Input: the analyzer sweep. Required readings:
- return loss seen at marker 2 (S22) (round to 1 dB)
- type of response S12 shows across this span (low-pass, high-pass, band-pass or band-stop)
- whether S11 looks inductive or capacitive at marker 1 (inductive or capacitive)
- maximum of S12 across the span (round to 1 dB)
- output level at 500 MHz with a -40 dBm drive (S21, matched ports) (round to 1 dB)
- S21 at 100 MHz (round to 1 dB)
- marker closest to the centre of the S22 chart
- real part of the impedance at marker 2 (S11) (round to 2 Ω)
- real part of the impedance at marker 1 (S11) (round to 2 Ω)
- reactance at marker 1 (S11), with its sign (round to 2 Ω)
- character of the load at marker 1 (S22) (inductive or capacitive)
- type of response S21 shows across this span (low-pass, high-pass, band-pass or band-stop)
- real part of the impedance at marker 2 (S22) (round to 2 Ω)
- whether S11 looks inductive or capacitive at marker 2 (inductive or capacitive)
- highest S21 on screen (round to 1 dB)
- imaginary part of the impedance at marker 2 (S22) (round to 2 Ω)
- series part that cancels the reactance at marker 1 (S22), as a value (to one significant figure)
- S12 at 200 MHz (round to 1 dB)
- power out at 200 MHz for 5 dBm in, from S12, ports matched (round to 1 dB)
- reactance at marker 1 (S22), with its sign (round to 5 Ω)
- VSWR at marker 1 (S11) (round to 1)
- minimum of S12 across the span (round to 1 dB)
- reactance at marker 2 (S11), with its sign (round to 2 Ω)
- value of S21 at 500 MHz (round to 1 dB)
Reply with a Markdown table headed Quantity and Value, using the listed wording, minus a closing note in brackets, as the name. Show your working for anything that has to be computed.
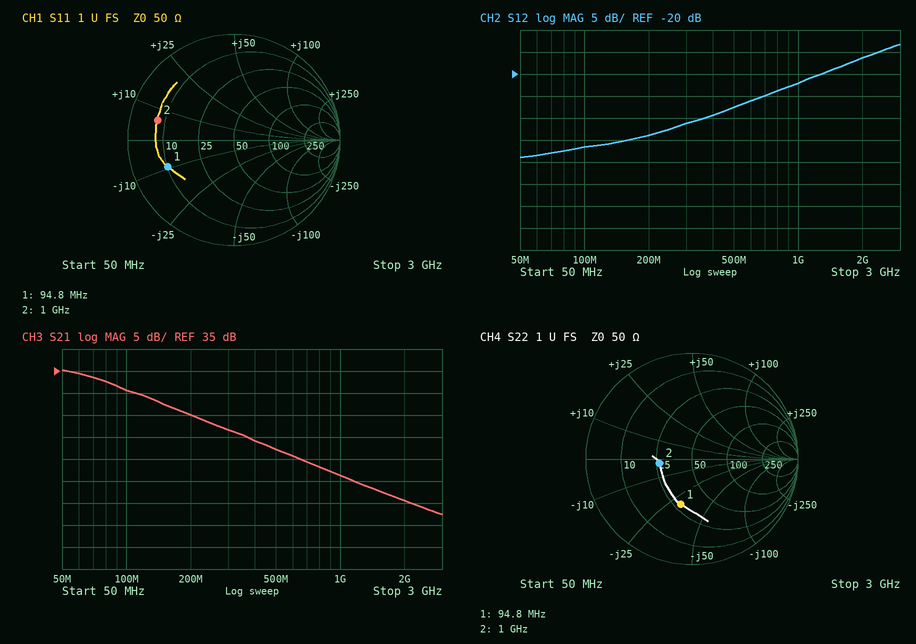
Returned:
| Quantity | Value |
|---|---|
| return loss seen at marker 2 (S22) | 10 dB |
| type of response S12 shows across this span | high-pass |
| whether S11 looks inductive or capacitive at marker 1 | capacitive |
| maximum of S12 across the span | -13 dB |
| output level at 500 MHz with a -40 dBm drive (S21, matched ports) | -40 dBm + (17 dB) = -23 dBm |
| S21 at 100 MHz | 31 dB |
| marker closest to the centre of the S22 chart | marker 2 |
| real part of the impedance at marker 2 (S11) | 8 Ω |
| real part of the impedance at marker 1 (S11) | 10 Ω |
| reactance at marker 1 (S11), with its sign | -10 Ω |
| character of the load at marker 1 (S22) | capacitive |
| type of response S21 shows across this span | low-pass |
| real part of the impedance at marker 2 (S22) | 26 Ω |
| whether S11 looks inductive or capacitive at marker 2 | inductive |
| highest S21 on screen | 35 dB |
| imaginary part of the impedance at marker 2 (S22) | -2 Ω |
| series part that cancels the reactance at marker 1 (S22), as a value | L = 30 Ω/(2π × 94.8 MHz) ≈ 50 nH |
| S12 at 200 MHz | -34 dB |
| power out at 200 MHz for 5 dBm in, from S12, ports matched | 5 dBm + (-34 dB) = -29 dBm |
| reactance at marker 1 (S22), with its sign | -30 Ω |
| VSWR at marker 1 (S11) | 5 |
| minimum of S12 across the span | -39 dB |
| reactance at marker 2 (S11), with its sign | +6 Ω |
| value of S21 at 500 MHz | 17 dB |
